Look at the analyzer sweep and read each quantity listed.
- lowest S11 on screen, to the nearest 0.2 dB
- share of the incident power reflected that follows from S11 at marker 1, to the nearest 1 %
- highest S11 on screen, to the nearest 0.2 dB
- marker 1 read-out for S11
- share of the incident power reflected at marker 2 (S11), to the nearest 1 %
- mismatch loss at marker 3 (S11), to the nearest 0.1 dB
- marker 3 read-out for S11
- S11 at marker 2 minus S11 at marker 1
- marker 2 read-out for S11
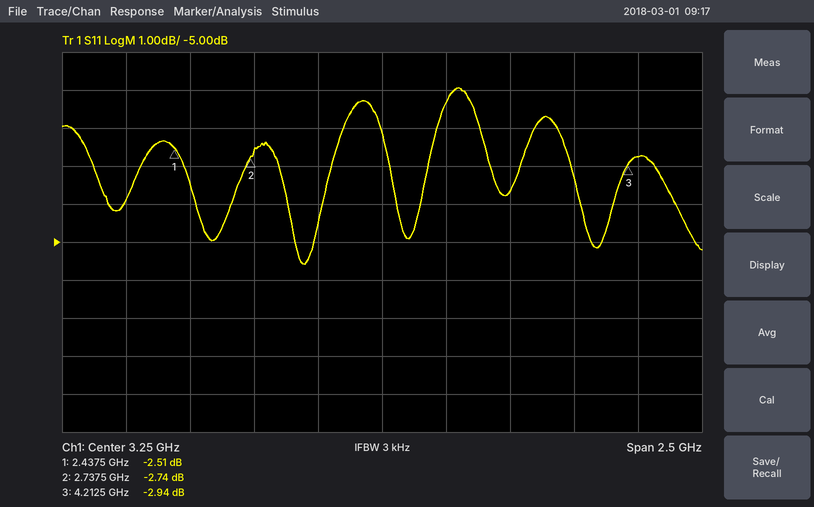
-5.6 dB
56 %
-1.0 dB
-2.51 dB
53 %
3.1 dB
-2.94 dB
-0.23 dB
-2.74 dB
